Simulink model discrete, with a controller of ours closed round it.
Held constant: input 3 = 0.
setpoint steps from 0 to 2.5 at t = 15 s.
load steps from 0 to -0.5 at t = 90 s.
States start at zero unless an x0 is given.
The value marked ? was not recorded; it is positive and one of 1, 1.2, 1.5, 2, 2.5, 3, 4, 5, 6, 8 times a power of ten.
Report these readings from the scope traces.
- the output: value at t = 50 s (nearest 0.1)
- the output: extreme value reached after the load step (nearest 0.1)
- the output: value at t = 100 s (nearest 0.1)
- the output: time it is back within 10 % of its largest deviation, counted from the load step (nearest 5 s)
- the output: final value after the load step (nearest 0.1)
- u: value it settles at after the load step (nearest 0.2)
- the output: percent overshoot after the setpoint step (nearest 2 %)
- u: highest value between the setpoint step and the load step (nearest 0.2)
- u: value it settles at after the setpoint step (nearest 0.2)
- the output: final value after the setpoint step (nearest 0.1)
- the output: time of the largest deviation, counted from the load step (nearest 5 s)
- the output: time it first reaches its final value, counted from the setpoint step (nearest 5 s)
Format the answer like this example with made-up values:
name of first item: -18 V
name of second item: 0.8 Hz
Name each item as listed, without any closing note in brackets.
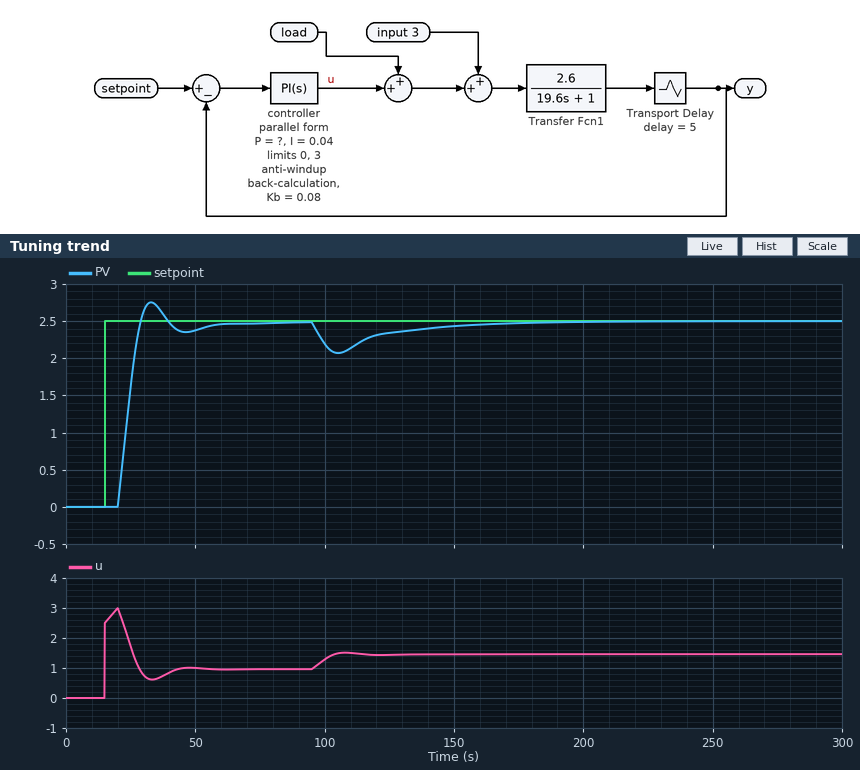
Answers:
the output: value at t = 50 s: 2.4
the output: extreme value reached after the load step: 2.1
the output: value at t = 100 s: 2.2
the output: time it is back within 10 % of its largest deviation, counted from the load step: 75 s
the output: final value after the load step: 2.5
u: value it settles at after the load step: 1.4
the output: percent overshoot after the setpoint step: 10 %
u: highest value between the setpoint step and the load step: 3.0
u: value it settles at after the setpoint step: 1.0
the output: final value after the setpoint step: 2.5
the output: time of the largest deviation, counted from the load step: 15 s
the output: time it first reaches its final value, counted from the setpoint step: 15 s
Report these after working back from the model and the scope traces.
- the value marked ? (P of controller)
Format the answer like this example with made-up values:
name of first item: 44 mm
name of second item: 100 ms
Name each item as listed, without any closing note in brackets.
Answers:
the value marked ?: 1
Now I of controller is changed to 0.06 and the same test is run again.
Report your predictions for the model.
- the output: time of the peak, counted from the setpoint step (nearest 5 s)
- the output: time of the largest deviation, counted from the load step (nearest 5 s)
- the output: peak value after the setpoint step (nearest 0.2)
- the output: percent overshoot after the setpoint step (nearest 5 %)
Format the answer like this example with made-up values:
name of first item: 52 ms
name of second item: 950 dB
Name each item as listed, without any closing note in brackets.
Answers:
the output: time of the peak, counted from the setpoint step: 20 s
the output: time of the largest deviation, counted from the load step: 15 s
the output: peak value after the setpoint step: 3.0
the output: percent overshoot after the setpoint step: 20 %
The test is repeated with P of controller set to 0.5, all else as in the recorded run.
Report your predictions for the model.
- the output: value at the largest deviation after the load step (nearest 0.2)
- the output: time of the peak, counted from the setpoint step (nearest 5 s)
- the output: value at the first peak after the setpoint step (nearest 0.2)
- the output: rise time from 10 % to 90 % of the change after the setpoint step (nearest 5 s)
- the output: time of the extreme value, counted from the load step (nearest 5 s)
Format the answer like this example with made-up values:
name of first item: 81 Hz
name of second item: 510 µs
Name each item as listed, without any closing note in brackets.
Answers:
the output: value at the largest deviation after the load step: 2.0
the output: time of the peak, counted from the setpoint step: 35 s
the output: value at the first peak after the setpoint step: 2.8
the output: rise time from 10 % to 90 % of the change after the setpoint step: 15 s
the output: time of the extreme value, counted from the load step: 20 s
